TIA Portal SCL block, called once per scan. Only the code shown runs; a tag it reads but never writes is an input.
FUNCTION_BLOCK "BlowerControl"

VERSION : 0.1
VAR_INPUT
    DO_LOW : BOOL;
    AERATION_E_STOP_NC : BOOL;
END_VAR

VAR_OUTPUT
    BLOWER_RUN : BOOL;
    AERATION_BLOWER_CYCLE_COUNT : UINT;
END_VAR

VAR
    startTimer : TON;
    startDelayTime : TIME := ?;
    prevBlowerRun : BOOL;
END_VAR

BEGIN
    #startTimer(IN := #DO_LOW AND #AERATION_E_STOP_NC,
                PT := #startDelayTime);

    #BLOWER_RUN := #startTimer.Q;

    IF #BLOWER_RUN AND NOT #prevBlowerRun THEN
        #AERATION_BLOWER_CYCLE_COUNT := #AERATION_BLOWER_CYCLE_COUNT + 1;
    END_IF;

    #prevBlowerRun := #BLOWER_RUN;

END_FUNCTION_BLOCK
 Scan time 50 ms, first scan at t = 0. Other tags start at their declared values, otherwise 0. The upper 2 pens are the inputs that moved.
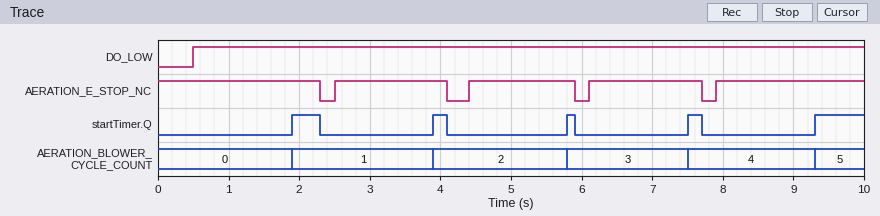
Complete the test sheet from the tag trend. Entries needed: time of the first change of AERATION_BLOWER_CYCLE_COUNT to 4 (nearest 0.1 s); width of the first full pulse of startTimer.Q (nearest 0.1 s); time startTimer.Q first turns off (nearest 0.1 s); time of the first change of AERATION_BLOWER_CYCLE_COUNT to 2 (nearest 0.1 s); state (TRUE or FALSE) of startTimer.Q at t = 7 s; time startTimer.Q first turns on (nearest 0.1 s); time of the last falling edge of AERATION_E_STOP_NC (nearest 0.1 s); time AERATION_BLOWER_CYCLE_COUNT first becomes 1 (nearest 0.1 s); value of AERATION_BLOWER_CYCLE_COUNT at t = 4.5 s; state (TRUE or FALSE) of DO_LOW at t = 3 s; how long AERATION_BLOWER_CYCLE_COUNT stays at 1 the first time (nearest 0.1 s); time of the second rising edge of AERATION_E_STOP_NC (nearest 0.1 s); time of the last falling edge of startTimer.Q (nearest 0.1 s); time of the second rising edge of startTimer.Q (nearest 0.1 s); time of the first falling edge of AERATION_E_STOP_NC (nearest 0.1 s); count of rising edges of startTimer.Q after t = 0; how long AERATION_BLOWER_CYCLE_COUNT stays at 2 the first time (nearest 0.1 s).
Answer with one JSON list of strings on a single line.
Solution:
["7.5 s", "0.4 s", "2.3 s", "3.9 s", "FALSE", "1.9 s", "7.7 s", "1.9 s", "2", "TRUE", "2.0 s", "4.4 s", "7.7 s", "3.9 s", "2.3 s", "5", "1.9 s"]
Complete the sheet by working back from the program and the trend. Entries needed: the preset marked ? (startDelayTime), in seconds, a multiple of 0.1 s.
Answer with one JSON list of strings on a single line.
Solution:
["1.4 s"]
